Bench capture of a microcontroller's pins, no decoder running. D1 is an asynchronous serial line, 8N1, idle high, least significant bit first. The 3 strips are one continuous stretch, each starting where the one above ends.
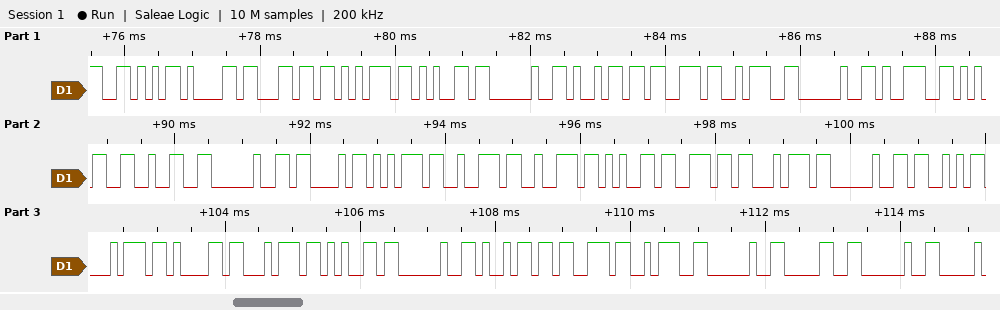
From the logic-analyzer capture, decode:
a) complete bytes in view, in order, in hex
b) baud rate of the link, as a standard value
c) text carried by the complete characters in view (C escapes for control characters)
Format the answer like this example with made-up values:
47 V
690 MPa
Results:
56 61 6C 75 65 20 69 73 3A 20 39 35 32 20 43 75 72 72 65 6E 74 20 53 74 61 74 65 20 69 73 3A 20 30 20
9600 baud
"Value is: 952 Current State is: 0 "
